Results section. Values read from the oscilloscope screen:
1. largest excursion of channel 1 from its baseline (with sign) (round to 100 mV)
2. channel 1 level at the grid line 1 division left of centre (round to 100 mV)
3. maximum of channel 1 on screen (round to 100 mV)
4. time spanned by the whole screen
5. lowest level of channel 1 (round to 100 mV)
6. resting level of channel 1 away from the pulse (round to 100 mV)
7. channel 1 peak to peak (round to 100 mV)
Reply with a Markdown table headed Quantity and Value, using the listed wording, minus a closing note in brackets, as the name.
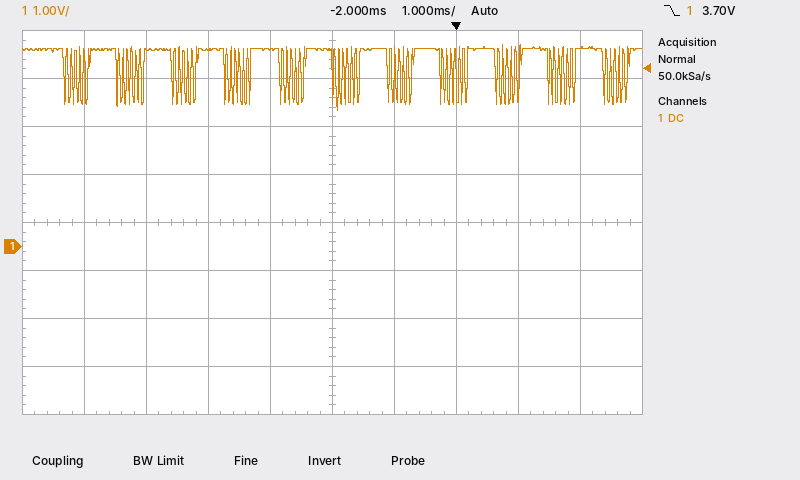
| Quantity | Value |
|---|---|
| largest excursion of channel 1 from its baseline (with sign) | -1.3 V |
| channel 1 level at the grid line 1 division left of centre | 4.1 V |
| maximum of channel 1 on screen | 4.2 V |
| time spanned by the whole screen | 10 ms |
| lowest level of channel 1 | 2.8 V |
| resting level of channel 1 away from the pulse | 4.1 V |
| channel 1 peak to peak | 1.4 V |
